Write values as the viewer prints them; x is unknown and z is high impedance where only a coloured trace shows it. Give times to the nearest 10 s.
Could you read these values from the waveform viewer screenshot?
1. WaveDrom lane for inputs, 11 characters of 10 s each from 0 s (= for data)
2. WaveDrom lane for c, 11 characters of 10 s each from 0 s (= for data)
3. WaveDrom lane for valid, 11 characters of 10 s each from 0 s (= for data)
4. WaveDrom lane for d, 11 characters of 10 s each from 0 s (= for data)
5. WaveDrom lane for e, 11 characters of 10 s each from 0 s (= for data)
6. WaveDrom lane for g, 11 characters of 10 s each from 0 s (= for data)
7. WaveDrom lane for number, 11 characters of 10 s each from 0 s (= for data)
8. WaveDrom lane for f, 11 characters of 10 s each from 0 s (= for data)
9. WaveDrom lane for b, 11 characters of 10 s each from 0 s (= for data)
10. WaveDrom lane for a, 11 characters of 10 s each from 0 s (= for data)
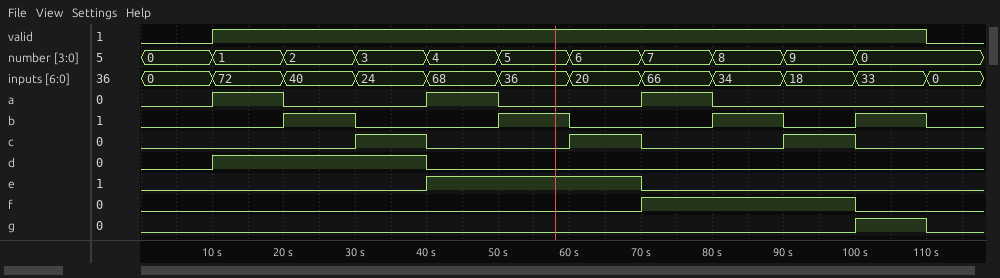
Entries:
{name: 'inputs', wave: '===========', data: '0 72 40 24 68 36 20 66 34 18 33'}
{name: 'c', wave: '0..10.10.10'}
{name: 'valid', wave: '01.........'}
{name: 'd', wave: '01..0......'}
{name: 'e', wave: '0...1..0...'}
{name: 'g', wave: '0.........1'}
{name: 'number', wave: '===========', data: '0 1 2 3 4 5 6 7 8 9 0'}
{name: 'f', wave: '0......1..0'}
{name: 'b', wave: '0.10.10.101'}
{name: 'a', wave: '010.10.10..'}
